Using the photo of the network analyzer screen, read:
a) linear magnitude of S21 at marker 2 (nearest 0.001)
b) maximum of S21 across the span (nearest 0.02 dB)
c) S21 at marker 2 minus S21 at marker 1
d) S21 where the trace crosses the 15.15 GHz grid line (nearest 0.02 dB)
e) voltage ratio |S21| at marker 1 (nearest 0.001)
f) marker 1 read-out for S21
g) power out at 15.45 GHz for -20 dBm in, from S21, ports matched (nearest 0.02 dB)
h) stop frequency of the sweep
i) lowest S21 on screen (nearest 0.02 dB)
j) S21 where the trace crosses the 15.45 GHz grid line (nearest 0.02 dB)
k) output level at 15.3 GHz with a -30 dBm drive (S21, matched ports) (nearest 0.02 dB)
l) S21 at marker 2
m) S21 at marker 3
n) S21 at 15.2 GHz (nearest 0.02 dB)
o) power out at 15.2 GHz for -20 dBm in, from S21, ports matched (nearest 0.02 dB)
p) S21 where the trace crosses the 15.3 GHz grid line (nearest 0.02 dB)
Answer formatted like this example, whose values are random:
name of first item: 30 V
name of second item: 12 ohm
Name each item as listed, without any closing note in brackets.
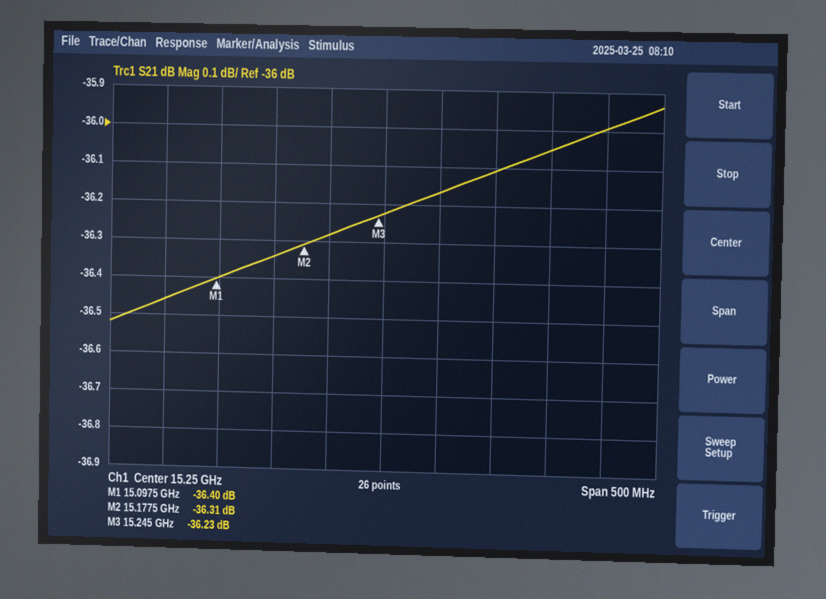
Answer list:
linear magnitude of S21 at marker 2: 0.015
maximum of S21 across the span: -35.94 dB
S21 at marker 2 minus S21 at marker 1: 0.09 dB
S21 where the trace crosses the 15.15 GHz grid line: -36.34 dB
voltage ratio |S21| at marker 1: 0.015
marker 1 read-out for S21: -36.40 dB
power out at 15.45 GHz for -20 dBm in, from S21, ports matched: -56.00 dBm
stop frequency of the sweep: 15.5 GHz
lowest S21 on screen: -36.52 dB
S21 where the trace crosses the 15.45 GHz grid line: -36.00 dB
output level at 15.3 GHz with a -30 dBm drive (S21, matched ports): -66.16 dBm
S21 at marker 2: -36.31 dB
S21 at marker 3: -36.23 dB
S21 at 15.2 GHz: -36.28 dB
power out at 15.2 GHz for -20 dBm in, from S21, ports matched: -56.28 dBm
S21 where the trace crosses the 15.3 GHz grid line: -36.16 dB
